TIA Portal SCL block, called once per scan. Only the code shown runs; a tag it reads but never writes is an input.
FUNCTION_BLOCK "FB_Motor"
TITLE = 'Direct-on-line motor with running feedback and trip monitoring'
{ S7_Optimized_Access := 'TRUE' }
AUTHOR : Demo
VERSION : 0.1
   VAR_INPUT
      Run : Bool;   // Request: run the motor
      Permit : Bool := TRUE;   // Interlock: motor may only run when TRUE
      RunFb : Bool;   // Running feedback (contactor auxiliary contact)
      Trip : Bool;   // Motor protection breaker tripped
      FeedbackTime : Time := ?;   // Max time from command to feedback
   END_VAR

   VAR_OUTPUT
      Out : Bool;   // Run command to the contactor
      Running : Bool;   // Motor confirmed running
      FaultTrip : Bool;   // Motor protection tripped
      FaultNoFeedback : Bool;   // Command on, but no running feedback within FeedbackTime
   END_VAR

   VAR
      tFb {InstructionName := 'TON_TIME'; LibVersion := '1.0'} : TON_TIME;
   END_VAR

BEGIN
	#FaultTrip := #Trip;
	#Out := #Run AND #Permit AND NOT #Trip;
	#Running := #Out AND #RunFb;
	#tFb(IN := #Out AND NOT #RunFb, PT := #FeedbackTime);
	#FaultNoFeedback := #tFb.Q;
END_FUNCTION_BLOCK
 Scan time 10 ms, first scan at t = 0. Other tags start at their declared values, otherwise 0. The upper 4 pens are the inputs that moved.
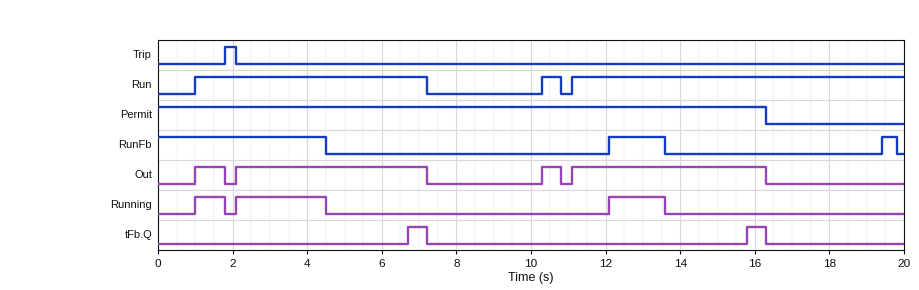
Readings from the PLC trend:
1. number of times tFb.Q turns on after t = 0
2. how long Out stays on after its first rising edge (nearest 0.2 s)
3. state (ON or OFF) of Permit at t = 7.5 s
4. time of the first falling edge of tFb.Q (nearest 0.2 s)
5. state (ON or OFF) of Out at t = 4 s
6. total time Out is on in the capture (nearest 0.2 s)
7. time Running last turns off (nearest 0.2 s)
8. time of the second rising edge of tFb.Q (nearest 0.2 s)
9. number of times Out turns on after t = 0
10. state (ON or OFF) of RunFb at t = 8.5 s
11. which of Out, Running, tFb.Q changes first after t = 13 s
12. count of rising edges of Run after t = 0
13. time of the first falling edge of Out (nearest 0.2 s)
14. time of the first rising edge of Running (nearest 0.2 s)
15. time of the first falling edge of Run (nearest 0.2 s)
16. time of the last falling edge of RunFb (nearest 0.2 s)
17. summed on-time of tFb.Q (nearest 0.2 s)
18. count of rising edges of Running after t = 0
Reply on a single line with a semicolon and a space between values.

2; 0.8 s; ON; 7.2 s; ON; 11.6 s; 13.6 s; 15.8 s; 4; OFF; Running; 3; 1.8 s; 1.0 s; 7.2 s; 19.8 s; 1.0 s; 3
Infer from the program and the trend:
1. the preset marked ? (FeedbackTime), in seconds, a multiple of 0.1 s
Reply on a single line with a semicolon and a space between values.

2.2 s
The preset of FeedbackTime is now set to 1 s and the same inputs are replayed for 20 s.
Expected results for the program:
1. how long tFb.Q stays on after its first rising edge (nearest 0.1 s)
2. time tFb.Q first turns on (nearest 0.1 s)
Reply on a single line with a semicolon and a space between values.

1.7 s; 5.5 s
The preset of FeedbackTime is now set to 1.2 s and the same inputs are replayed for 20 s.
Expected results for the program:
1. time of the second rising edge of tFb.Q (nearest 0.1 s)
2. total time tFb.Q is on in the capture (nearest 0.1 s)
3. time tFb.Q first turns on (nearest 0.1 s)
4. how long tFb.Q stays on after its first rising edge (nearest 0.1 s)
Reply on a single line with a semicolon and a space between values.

14.8 s; 3.0 s; 5.7 s; 1.5 s
